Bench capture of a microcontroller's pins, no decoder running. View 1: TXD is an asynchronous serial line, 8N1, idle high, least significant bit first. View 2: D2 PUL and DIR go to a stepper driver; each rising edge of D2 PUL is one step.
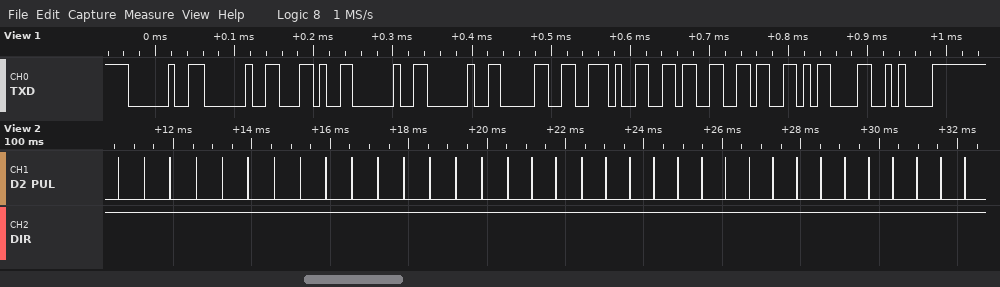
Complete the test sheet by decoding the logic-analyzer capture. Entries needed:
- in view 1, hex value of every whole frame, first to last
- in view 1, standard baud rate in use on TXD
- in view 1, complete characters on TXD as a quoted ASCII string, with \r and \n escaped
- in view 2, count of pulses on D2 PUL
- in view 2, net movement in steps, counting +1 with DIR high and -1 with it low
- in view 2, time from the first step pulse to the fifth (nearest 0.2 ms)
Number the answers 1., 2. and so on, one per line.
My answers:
1. 20 20 2C 20 20 30 2E 36 36 0D 0A
2. 115200 baud
3. "  ,  0.66\r\n"
4. 35
5. +35
6. 2.6 ms
